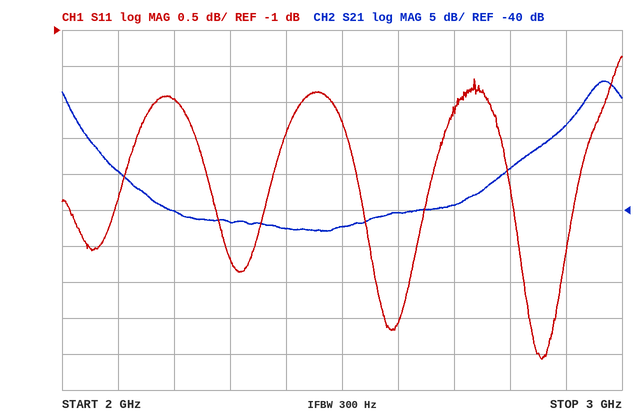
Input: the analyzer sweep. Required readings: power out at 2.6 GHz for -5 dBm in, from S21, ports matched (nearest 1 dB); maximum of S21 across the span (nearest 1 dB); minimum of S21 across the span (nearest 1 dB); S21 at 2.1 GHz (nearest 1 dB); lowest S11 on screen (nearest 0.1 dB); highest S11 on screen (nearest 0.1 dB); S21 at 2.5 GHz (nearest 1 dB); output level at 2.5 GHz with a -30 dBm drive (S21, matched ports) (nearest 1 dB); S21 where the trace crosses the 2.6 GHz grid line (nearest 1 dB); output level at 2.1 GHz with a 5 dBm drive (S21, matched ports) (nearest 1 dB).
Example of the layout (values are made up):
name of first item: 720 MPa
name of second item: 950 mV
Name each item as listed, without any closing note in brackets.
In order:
power out at 2.6 GHz for -5 dBm in, from S21, ports matched: -45 dBm
maximum of S21 across the span: -22 dB
minimum of S21 across the span: -43 dB
S21 at 2.1 GHz: -35 dB
lowest S11 on screen: -5.6 dB
highest S11 on screen: -1.4 dB
S21 at 2.5 GHz: -42 dB
output level at 2.5 GHz with a -30 dBm drive (S21, matched ports): -72 dBm
S21 where the trace crosses the 2.6 GHz grid line: -40 dB
output level at 2.1 GHz with a 5 dBm drive (S21, matched ports): -30 dBm
